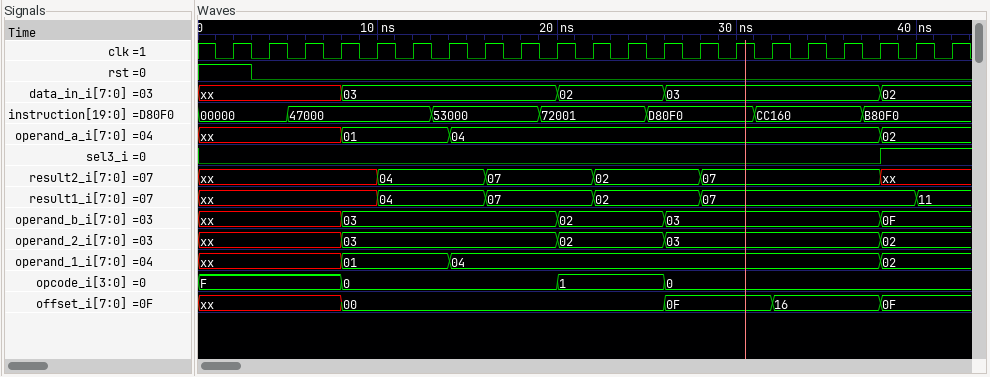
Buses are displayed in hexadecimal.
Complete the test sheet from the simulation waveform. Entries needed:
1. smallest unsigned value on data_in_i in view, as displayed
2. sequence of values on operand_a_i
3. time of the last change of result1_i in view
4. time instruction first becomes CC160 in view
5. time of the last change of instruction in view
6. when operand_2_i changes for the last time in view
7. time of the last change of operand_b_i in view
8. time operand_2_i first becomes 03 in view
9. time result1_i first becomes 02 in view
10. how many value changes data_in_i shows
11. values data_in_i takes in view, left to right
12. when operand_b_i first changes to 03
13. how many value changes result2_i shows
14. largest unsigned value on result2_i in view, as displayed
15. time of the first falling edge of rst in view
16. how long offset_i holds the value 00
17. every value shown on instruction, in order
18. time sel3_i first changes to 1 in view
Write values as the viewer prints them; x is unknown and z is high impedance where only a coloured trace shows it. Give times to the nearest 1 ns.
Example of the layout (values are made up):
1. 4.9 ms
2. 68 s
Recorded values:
1. 02
2. xx, 01, 04, 02
3. 40 ns
4. 31 ns
5. 37 ns
6. 38 ns
7. 38 ns
8. 8 ns
9. 22 ns
10. 4
11. xx, 03, 02, 03, 02
12. 8 ns
13. 5
14. 07
15. 3 ns
16. 18 ns
17. 00000, 47000, 53000, 72001, D80F0, CC160, B80F0
18. 38 ns
